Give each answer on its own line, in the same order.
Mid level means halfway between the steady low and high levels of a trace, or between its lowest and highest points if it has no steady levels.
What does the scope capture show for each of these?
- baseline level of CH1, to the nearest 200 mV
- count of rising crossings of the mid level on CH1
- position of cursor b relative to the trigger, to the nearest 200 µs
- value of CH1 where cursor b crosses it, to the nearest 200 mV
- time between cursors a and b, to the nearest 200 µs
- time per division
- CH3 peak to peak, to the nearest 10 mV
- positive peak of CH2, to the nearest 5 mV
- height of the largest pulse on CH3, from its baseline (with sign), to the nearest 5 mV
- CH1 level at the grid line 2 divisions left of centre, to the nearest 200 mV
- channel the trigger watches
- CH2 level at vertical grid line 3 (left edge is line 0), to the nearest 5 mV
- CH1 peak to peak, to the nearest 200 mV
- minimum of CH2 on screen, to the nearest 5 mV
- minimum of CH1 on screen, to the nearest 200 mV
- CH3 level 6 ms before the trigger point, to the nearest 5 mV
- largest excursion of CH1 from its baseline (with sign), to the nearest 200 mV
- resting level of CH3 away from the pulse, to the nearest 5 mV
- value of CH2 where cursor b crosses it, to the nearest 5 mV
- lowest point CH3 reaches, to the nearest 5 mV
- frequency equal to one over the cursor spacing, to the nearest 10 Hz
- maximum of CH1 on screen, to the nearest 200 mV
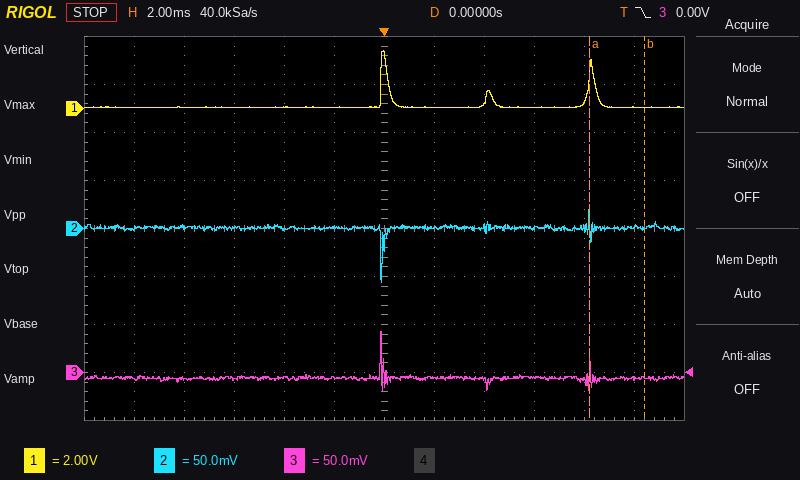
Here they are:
0.0 V
2
+10.4 ms
0.0 V
2.2 ms
2 ms
60 mV
20 mV
+50 mV
0.0 V
CH3
0 mV
2.4 V
-55 mV
0.0 V
-5 mV
+2.4 V
-5 mV
0 mV
-20 mV
450 Hz
2.4 V
